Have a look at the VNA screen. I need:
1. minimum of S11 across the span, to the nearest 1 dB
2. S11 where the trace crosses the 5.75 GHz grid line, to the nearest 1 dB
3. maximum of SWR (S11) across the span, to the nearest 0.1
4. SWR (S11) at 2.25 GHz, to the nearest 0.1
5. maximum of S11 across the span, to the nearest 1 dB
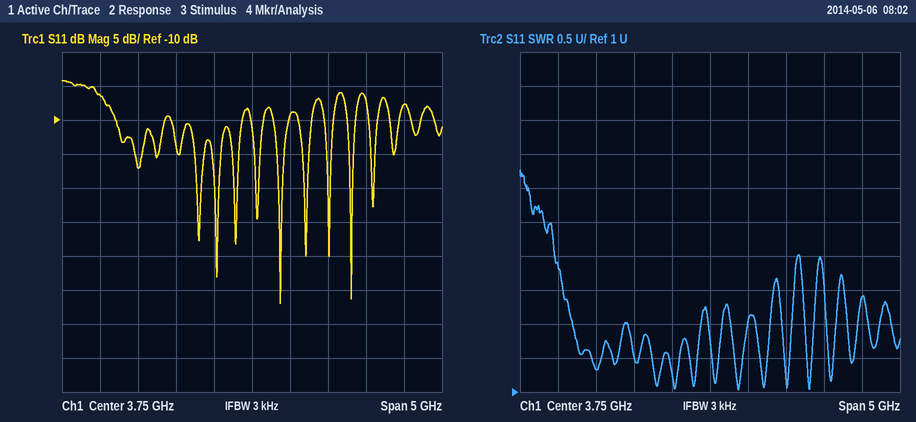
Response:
-37 dB
-8 dB
4.3
1.3
-4 dB
